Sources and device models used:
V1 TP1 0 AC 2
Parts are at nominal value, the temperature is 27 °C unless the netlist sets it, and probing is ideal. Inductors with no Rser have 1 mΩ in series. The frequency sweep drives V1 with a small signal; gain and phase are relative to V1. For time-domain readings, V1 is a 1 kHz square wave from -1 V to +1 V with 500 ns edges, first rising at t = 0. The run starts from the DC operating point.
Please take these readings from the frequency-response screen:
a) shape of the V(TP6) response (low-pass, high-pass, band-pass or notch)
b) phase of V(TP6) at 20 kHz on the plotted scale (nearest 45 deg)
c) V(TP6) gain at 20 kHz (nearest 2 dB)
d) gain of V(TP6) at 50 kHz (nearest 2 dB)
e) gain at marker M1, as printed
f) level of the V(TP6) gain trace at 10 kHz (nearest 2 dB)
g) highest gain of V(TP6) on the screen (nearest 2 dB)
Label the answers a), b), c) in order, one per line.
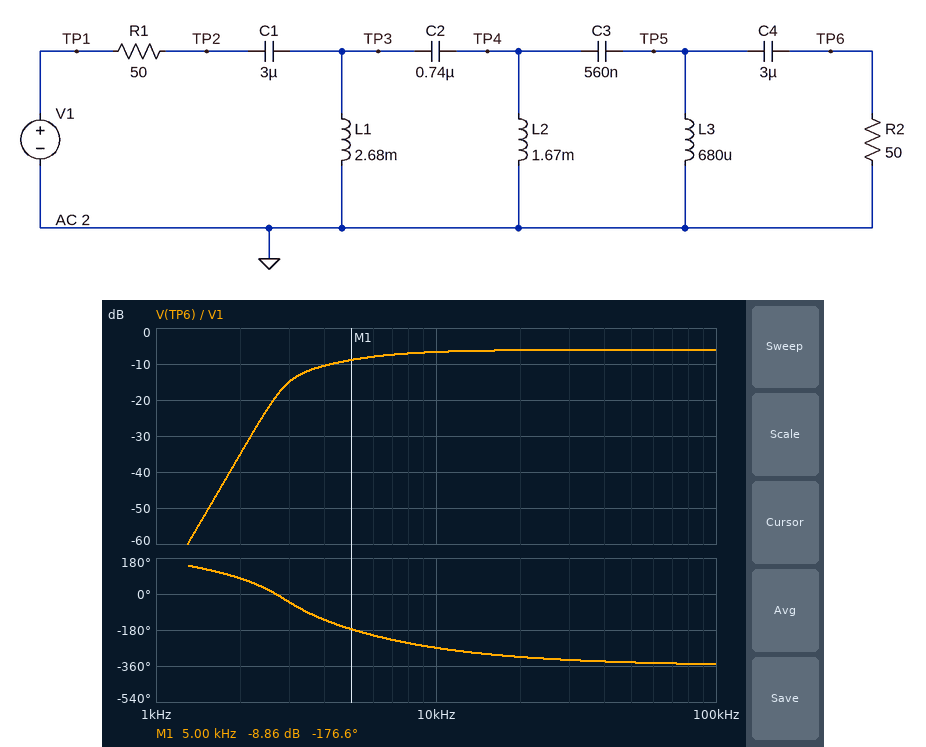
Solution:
a) high-pass
b) -315 deg
c) -6 dB
d) -6 dB
e) -8.86 dB
f) -6 dB
g) -6 dB
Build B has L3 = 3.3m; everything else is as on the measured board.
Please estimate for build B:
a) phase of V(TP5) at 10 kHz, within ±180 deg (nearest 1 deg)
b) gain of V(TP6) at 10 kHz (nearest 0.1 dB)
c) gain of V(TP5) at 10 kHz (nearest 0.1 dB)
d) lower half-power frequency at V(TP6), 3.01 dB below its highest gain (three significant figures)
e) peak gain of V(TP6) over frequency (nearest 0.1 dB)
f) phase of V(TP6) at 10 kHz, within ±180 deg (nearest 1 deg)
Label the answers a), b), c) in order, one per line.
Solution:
a) 58 deg
b) -6.1 dB
c) -6.0 dB
d) 2.64 kHz
e) -6.0 dB
f) 64 deg
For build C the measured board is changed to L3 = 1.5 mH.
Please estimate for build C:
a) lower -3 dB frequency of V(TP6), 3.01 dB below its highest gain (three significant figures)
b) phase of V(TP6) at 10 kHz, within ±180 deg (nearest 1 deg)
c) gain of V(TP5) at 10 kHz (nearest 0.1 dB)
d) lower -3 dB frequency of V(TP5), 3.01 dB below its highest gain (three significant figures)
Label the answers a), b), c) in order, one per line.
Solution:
a) 2.87 kHz
b) 73 deg
c) -6.0 dB
d) 2.81 kHz
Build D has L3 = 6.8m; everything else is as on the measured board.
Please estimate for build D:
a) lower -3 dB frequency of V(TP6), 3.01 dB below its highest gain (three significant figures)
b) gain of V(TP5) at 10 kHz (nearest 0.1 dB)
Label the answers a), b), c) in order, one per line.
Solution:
a) 2.81 kHz
b) -6.1 dB
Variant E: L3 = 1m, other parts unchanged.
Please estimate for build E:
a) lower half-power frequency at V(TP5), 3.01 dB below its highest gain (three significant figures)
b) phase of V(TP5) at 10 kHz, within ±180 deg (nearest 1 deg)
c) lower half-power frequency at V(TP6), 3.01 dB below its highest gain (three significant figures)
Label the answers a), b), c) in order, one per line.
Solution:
a) 3.29 kHz
b) 75 deg
c) 3.42 kHz
